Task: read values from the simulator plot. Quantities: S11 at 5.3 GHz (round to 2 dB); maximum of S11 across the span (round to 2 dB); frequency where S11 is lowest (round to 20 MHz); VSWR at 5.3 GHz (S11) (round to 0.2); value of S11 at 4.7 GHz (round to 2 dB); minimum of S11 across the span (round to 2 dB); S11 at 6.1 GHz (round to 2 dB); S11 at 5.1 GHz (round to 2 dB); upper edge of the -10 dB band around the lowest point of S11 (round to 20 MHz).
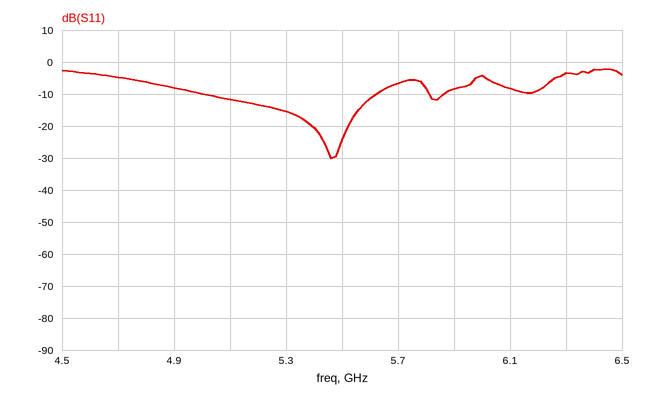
-16 dB
-2 dB
5.46 GHz
1.4
-4 dB
-30 dB
-8 dB
-12 dB
5.62 GHz
